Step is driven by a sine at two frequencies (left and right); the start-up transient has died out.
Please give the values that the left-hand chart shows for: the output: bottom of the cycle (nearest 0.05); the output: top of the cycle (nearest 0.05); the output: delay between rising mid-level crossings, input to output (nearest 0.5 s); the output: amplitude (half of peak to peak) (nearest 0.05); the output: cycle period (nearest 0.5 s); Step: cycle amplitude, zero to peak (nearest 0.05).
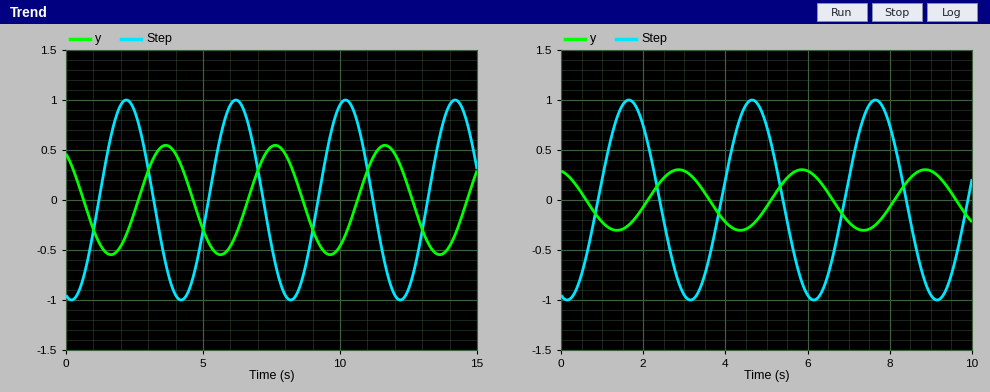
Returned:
-0.55
0.55
1.5 s
0.55
4.0 s
1.00
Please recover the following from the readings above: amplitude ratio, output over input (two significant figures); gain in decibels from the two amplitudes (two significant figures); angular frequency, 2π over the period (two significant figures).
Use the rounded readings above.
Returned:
0.55
-5.2 dB
1.6 rad/s
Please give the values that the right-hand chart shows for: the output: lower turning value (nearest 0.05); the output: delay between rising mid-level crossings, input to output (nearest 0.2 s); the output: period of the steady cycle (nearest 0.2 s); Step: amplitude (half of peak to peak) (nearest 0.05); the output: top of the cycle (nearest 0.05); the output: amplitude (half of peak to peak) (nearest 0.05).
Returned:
-0.30
1.2 s
3.0 s
1.00
0.30
0.30
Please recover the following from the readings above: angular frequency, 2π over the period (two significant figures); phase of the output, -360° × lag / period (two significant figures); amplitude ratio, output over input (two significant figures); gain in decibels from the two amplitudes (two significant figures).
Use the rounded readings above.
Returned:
2.1 rad/s
-140°
0.30
-10 dB
